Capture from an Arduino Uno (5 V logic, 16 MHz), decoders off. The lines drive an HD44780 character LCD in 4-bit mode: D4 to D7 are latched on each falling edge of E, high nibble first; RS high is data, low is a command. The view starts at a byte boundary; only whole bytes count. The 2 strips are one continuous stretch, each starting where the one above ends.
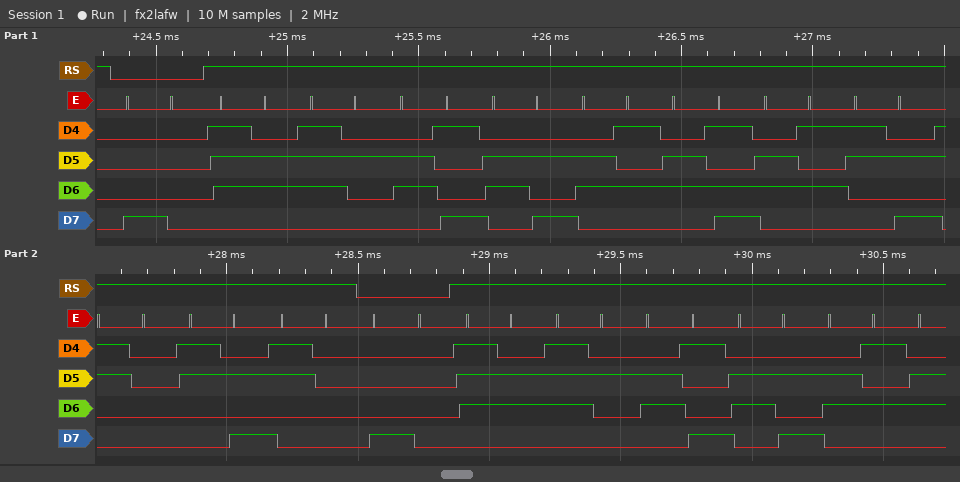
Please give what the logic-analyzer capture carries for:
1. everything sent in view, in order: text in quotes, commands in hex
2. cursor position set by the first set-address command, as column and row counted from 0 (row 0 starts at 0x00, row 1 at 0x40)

0x80 "vrijeme:0:0" 0x80 "vrije"
column 0, row 0
